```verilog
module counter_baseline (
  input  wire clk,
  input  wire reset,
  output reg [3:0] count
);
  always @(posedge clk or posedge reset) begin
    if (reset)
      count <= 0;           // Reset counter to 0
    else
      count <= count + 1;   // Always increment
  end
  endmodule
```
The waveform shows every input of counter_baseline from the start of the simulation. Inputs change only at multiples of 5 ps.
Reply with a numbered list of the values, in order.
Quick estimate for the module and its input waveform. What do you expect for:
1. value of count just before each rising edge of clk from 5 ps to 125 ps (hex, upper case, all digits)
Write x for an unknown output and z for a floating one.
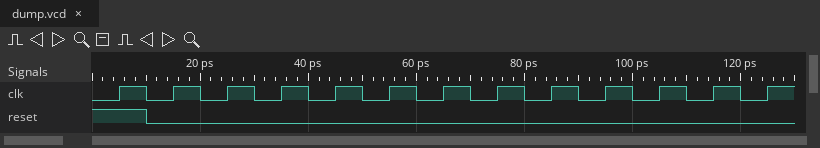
1. 0, 0, 1, 2, 3, 4, 5, 6, 7, 8, 9, A, B
